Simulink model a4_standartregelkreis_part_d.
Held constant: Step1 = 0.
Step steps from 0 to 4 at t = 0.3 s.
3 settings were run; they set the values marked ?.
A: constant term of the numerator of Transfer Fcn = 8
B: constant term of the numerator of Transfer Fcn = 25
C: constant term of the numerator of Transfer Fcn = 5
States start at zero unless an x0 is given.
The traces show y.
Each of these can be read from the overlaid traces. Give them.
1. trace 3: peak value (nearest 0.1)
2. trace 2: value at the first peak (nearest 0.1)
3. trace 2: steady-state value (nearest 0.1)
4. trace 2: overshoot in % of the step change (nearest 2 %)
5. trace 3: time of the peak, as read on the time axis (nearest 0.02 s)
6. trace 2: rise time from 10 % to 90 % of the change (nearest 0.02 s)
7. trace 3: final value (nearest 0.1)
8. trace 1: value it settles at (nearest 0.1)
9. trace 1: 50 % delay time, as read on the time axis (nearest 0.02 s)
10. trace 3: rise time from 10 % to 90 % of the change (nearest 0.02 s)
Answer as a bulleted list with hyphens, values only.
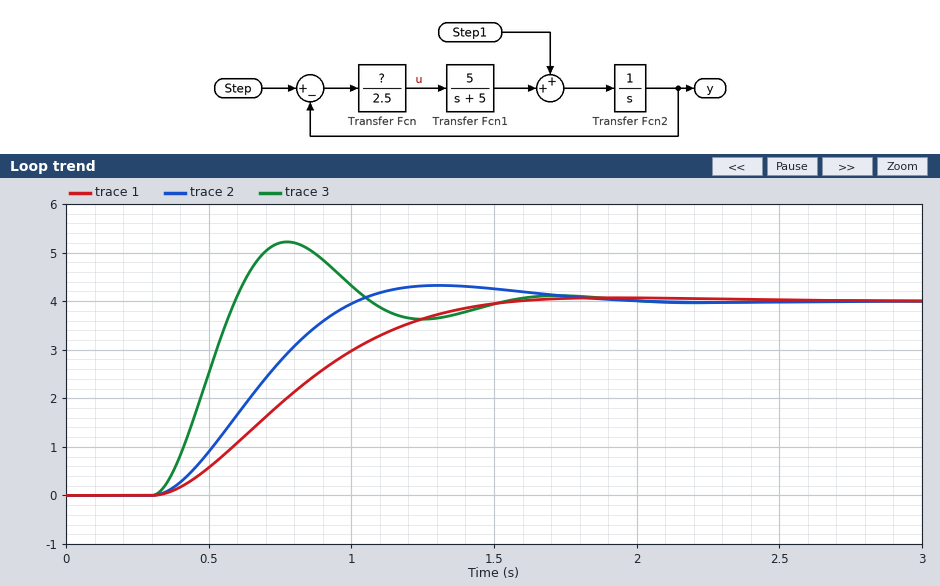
- 5.2
- 4.3
- 4.0
- 8 %
- 0.78 s
- 0.48 s
- 4.0
- 4.0
- 0.78 s
- 0.20 s
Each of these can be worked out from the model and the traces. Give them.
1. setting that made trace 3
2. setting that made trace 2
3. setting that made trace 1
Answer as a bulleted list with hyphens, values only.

- B
- A
- C
